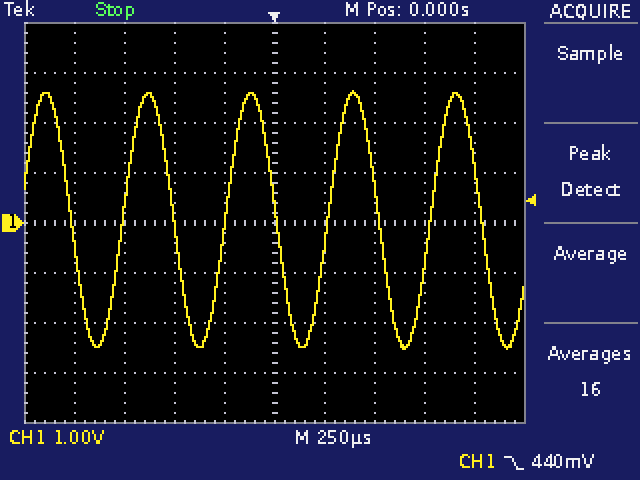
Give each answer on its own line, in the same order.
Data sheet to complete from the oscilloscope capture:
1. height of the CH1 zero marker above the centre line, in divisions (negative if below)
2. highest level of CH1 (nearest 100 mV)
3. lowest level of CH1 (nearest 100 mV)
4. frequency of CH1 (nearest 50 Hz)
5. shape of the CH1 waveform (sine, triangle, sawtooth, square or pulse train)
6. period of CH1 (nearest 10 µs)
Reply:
0.0 div
2.6 V
-2.5 V
1.95 kHz
sine
510 µs
